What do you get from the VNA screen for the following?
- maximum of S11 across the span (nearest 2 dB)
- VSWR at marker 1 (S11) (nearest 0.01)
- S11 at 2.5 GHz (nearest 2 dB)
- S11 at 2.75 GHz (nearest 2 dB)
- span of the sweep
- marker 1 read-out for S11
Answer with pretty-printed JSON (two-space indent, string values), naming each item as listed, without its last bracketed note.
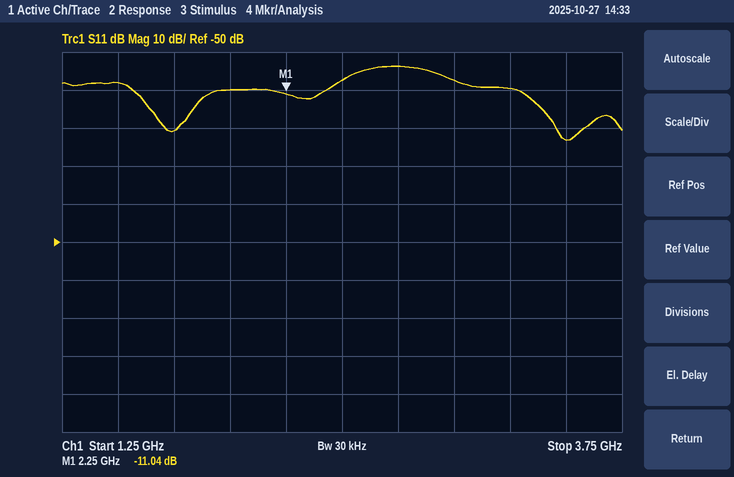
{
  "maximum of S11 across the span": "-4 dB",
  "VSWR at marker 1 (S11)": "1.78",
  "S11 at 2.5 GHz": "-8 dB",
  "S11 at 2.75 GHz": "-4 dB",
  "span of the sweep": "2.5 GHz",
  "marker 1 read-out for S11": "-11.04 dB"
}
